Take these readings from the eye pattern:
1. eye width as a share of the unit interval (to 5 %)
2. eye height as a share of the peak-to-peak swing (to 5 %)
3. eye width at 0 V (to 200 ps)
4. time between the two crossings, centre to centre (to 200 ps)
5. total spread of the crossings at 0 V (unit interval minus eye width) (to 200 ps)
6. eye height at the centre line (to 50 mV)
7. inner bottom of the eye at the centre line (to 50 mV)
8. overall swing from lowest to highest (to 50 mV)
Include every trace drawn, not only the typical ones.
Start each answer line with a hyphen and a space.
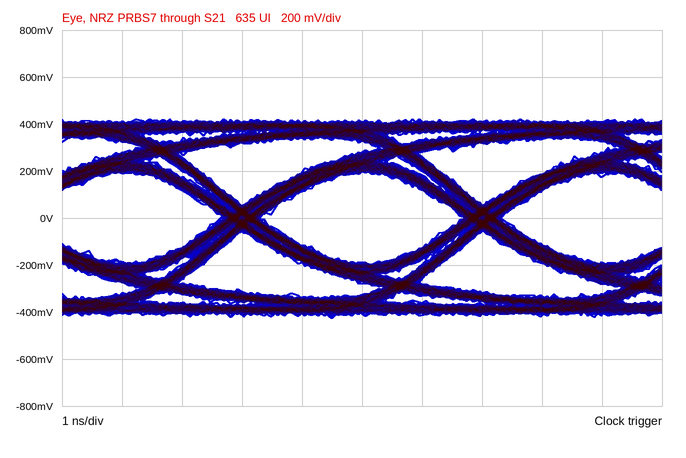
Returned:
- 85 %
- 45 %
- 3.4 ns
- 4.0 ns
- 600 ps
- 400 mV
- -200 mV
- 850 mV
